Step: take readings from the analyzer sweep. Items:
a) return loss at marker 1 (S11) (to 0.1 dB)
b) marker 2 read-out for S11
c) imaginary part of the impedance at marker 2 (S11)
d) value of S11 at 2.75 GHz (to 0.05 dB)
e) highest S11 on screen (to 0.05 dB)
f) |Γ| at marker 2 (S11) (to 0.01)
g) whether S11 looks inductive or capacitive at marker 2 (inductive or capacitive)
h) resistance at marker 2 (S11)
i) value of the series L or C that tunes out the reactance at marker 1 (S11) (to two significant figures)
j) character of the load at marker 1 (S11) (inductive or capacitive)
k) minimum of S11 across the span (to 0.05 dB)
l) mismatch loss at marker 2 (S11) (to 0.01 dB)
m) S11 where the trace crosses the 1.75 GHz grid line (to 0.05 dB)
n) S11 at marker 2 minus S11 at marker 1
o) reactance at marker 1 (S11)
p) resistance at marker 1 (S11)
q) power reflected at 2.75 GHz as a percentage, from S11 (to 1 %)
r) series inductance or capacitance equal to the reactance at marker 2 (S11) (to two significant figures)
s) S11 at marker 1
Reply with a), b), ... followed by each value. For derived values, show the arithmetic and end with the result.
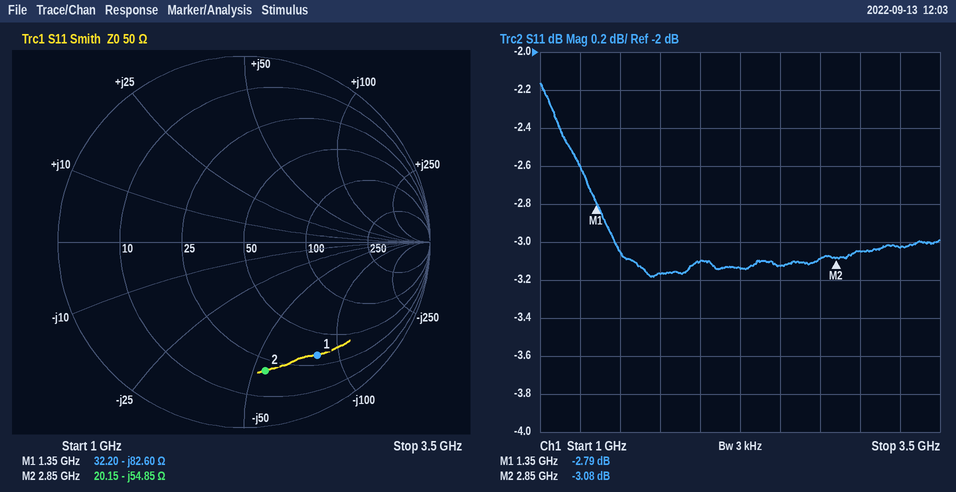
a) 2.8 dB
b) -3.08 dB
c) -54.85 Ω
d) -3.10 dB
e) -2.15 dB
f) 0.70
g) capacitive
h) 20.15 Ω
i) L = 82.6 Ω/(2π × 1.35 GHz) ≈ 9.7 nH
j) capacitive
k) -3.20 dB
l) −10 log10(1 − 10^(-3.08/10)) ≈ 2.94 dB
m) -3.15 dB
n) -3.08 − (-2.79) = -0.29 dB
o) -82.60 Ω
p) 32.20 Ω
q) 10^(-3.1/10) ≈ 49 %
r) C = 1/(2π × 2.85 GHz × 54.85 Ω) ≈ 1.0 pF
s) -2.79 dB
